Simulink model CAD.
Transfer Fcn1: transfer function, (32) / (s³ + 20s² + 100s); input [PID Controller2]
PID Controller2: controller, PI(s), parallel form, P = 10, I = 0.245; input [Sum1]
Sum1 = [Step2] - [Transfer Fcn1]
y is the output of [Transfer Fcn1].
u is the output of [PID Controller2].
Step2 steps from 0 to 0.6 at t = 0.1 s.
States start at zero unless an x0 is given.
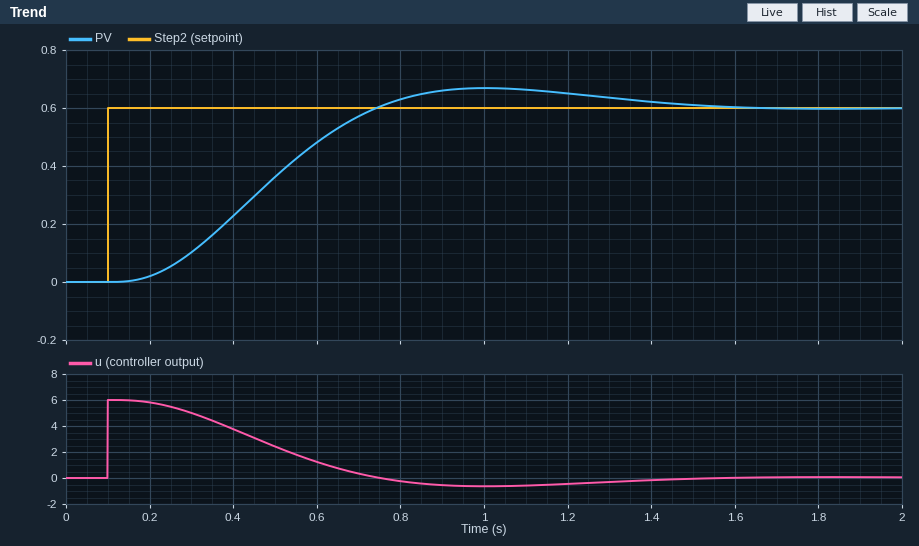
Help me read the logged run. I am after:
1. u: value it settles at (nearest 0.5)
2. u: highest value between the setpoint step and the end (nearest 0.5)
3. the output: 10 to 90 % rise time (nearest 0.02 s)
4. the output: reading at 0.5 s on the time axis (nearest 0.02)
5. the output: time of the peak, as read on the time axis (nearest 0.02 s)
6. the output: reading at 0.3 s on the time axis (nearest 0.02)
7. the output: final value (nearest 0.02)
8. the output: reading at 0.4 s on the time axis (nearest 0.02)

0.0
6.0
0.40 s
0.36
1.00 s
0.10
0.60
0.22
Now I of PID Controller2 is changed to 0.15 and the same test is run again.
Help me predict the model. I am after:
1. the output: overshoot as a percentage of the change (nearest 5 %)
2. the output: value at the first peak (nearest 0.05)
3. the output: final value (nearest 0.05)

10 %
0.65
0.60
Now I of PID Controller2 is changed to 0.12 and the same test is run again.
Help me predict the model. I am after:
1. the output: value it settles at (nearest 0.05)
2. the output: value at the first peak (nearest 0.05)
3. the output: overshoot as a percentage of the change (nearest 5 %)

0.60
0.65
10 %
